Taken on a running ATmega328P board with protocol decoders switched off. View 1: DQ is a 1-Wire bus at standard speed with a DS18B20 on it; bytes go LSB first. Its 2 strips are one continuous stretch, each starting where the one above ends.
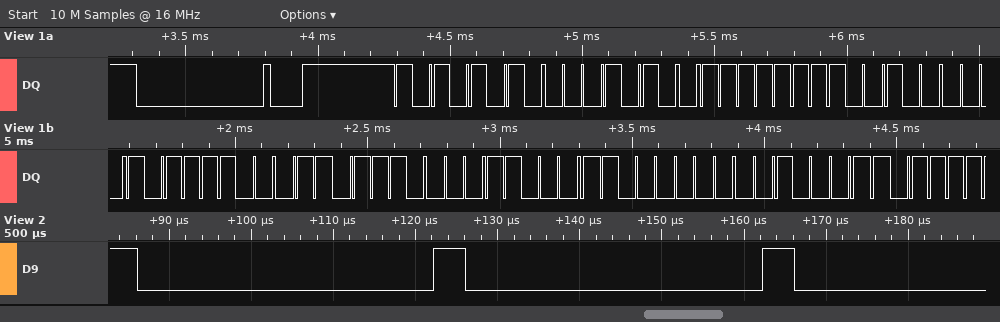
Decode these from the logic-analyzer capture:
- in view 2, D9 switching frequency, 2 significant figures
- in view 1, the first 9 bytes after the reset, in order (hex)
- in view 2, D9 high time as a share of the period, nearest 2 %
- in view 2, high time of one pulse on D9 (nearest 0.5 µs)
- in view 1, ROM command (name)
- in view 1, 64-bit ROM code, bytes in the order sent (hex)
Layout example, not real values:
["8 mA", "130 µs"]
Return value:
["25 kHz", "55 28 FF 04 3D 76 18 03 C4", "10 %", "4.0 µs", "Match ROM", "28 FF 04 3D 76 18 03 C4"]
